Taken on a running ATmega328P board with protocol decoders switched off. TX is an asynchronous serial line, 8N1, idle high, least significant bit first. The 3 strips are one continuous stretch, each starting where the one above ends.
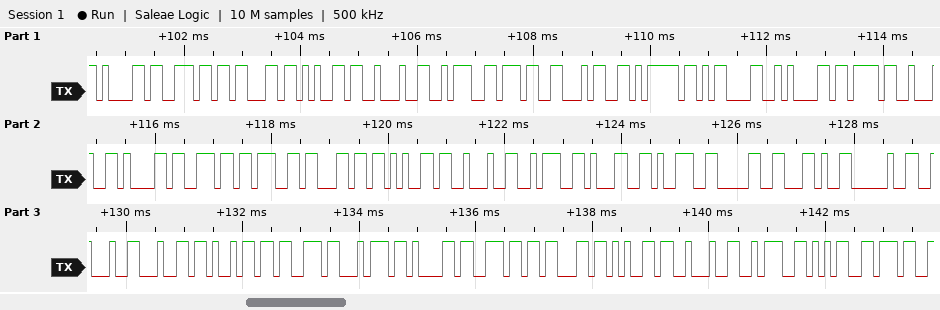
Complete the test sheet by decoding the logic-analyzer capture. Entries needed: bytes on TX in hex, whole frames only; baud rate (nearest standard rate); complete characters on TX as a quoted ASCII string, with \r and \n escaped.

0x61 0x6E 0x63 0x65 0x22 0x3A 0x37 0x34 0x7D 0x0D 0x0A 0x7B 0x22 0x61 0x6E 0x67 0x6C 0x65 0x22 0x3A 0x31 0x39 0x30 0x2C 0x20 0x22 0x64 0x69 0x73 0x74 0x61 0x6E 0x63 0x65 0x22 0x3A 0x35 0x37
9600 baud
"ance\":74}\r\n{\"angle\":190, \"distance\":57"
